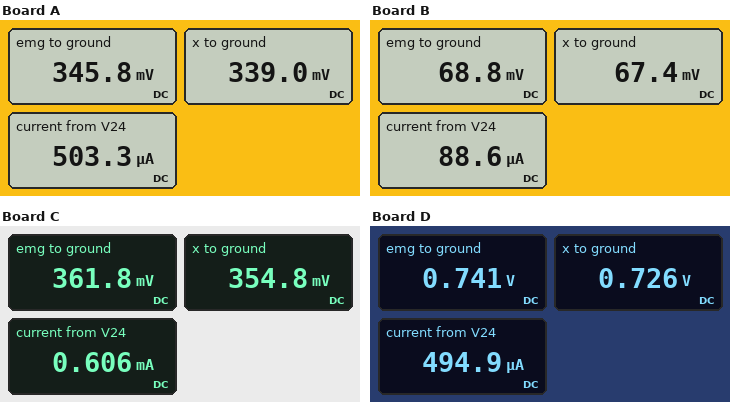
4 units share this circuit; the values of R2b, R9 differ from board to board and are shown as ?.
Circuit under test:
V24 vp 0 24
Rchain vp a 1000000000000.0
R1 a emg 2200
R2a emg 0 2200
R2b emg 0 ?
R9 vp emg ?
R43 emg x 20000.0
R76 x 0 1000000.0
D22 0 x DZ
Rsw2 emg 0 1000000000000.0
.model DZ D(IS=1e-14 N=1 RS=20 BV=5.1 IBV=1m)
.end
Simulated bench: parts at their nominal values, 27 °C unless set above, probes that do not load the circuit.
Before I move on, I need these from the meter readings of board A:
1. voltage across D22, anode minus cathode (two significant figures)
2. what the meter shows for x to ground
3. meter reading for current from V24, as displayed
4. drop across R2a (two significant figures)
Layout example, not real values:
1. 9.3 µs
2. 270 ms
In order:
1. -340 mV
2. 339.0 mV
3. 503.3 µA
4. 350 mV
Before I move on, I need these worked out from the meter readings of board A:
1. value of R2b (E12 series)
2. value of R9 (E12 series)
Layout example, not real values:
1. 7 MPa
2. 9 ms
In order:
1. 1 kΩ
2. 47 kΩ
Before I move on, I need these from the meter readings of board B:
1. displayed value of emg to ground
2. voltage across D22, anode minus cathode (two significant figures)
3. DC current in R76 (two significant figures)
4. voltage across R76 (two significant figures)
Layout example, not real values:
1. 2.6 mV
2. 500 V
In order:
1. 68.8 mV
2. -67 mV
3. 67 nA
4. 67 mV
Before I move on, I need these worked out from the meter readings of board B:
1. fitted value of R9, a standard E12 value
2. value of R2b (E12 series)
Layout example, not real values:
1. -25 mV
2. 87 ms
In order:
1. 270 kΩ
2. 1.2 kΩ
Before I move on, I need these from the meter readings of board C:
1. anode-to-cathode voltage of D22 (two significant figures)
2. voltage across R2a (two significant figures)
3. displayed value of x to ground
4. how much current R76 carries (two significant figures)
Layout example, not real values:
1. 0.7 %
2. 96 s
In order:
1. -350 mV
2. 360 mV
3. 354.8 mV
4. 350 nA
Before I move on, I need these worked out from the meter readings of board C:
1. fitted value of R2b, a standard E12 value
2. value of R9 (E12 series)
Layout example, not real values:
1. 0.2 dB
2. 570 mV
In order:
1. 820 Ω
2. 39 kΩ
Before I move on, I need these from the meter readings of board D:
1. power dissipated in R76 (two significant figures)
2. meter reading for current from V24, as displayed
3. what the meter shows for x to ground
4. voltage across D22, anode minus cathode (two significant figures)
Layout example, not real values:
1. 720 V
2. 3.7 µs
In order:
1. 530 nW
2. 494.9 µA
3. 0.726 V
4. -730 mV
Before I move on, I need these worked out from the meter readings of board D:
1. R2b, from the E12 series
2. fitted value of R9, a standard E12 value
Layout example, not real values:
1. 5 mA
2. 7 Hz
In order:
1. 4.7 kΩ
2. 47 kΩ
